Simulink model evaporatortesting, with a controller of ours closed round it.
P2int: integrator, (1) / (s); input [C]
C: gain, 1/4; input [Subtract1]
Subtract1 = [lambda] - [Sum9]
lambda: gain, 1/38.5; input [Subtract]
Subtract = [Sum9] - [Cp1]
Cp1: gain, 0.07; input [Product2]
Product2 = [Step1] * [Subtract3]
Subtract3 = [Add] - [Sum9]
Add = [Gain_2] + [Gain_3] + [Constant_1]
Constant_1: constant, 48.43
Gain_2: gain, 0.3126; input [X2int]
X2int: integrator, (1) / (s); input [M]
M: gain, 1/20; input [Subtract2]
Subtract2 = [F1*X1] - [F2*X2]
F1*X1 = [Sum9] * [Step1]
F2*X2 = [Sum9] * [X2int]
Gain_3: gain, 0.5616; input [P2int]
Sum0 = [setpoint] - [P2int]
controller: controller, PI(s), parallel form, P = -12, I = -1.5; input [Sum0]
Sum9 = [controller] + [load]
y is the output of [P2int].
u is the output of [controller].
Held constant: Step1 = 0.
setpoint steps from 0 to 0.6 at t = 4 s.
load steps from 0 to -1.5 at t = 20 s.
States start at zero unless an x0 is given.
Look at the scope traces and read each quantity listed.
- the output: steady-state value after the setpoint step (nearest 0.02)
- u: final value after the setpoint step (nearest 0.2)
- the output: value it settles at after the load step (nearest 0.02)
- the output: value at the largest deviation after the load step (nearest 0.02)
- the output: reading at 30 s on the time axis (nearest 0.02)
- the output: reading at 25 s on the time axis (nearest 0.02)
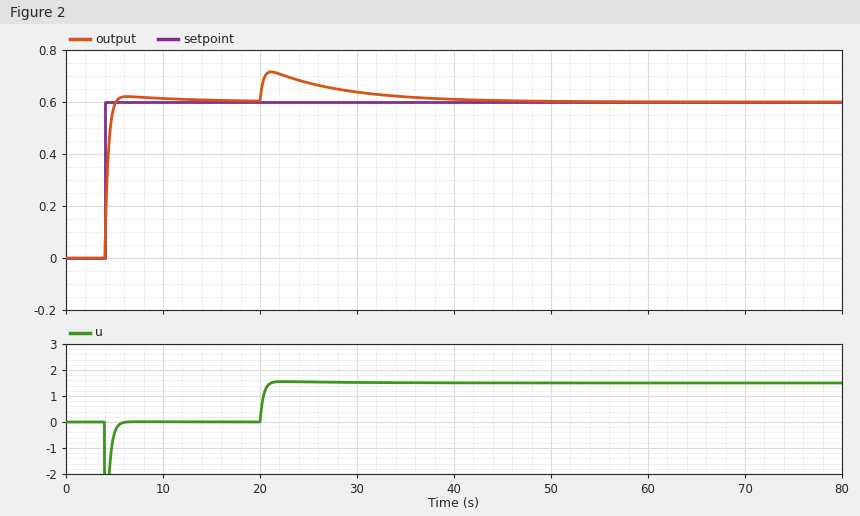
0.60
0.0
0.60
0.72
0.64
0.68
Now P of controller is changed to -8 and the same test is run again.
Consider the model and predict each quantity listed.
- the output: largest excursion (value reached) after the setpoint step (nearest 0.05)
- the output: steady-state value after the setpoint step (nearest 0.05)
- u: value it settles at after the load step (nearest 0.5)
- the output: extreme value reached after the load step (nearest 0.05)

0.65
0.60
1.5
0.75
